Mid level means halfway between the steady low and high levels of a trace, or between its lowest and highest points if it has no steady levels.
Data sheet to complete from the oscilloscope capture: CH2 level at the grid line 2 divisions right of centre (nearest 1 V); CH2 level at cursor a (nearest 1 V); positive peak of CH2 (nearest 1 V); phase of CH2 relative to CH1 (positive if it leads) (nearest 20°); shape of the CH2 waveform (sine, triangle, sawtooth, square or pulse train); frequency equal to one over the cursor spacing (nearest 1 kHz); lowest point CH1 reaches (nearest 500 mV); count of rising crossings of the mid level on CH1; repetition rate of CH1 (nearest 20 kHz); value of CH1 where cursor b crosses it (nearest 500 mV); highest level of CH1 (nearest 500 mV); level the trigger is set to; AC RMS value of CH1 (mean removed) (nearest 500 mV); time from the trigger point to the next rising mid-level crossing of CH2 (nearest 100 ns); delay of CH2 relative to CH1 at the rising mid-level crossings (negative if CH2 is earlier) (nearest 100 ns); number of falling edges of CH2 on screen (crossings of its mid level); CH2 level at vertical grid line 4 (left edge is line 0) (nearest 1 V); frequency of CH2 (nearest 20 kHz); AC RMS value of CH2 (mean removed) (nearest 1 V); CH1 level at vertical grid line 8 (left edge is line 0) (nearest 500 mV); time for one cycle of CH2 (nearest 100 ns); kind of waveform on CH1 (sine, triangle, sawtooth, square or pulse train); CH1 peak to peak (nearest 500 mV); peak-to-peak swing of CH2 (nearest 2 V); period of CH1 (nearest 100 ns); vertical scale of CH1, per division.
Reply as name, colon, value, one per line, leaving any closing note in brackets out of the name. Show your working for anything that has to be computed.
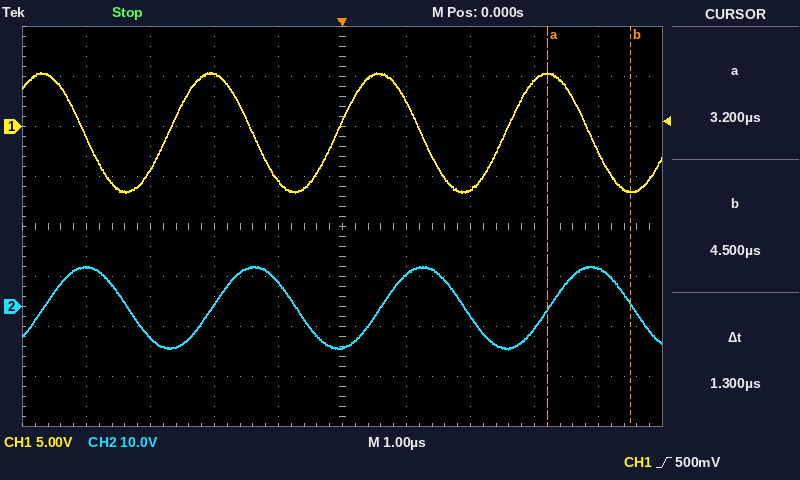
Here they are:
CH2 level at the grid line 2 divisions right of centre: -2 V
CH2 level at cursor a: -1 V
positive peak of CH2: 8 V
phase of CH2 relative to CH1 (positive if it leads): −360° × (+700 ns) / 2.6 µs ≈ -96.9°, so -100° to the nearest 20°
shape of the CH2 waveform: sine
frequency equal to one over the cursor spacing: 1 / 1.3 µs ≈ 769 kHz
lowest point CH1 reaches: -6.5 V
count of rising crossings of the mid level on CH1: 3
repetition rate of CH1: 1 / 2.6 µs ≈ 385 kHz, so 380 kHz to the nearest 20 kHz
value of CH1 where cursor b crosses it: -6.5 V
highest level of CH1: 5.5 V
level the trigger is set to: 500 mV
AC RMS value of CH1 (mean removed): 12.0 V / (2√2) ≈ 4.24 V, so 4.0 V to the nearest 500 mV
time from the trigger point to the next rising mid-level crossing of CH2: 600 ns
delay of CH2 relative to CH1 at the rising mid-level crossings (negative if CH2 is earlier): +700 ns
number of falling edges of CH2 on screen: 4
CH2 level at vertical grid line 4 (left edge is line 0): 5 V
frequency of CH2: 1 / 2.6 µs ≈ 385 kHz, so 380 kHz to the nearest 20 kHz
AC RMS value of CH2 (mean removed): 16 V / (2√2) ≈ 6 V
CH1 level at vertical grid line 8 (left edge is line 0): 4.5 V
time for one cycle of CH2: 2.6 µs
kind of waveform on CH1: sine
CH1 peak to peak: 5.5 V − (-6.5 V) = 12.0 V
peak-to-peak swing of CH2: 16 V
period of CH1: 2.6 µs
vertical scale of CH1, per division: 5 V
